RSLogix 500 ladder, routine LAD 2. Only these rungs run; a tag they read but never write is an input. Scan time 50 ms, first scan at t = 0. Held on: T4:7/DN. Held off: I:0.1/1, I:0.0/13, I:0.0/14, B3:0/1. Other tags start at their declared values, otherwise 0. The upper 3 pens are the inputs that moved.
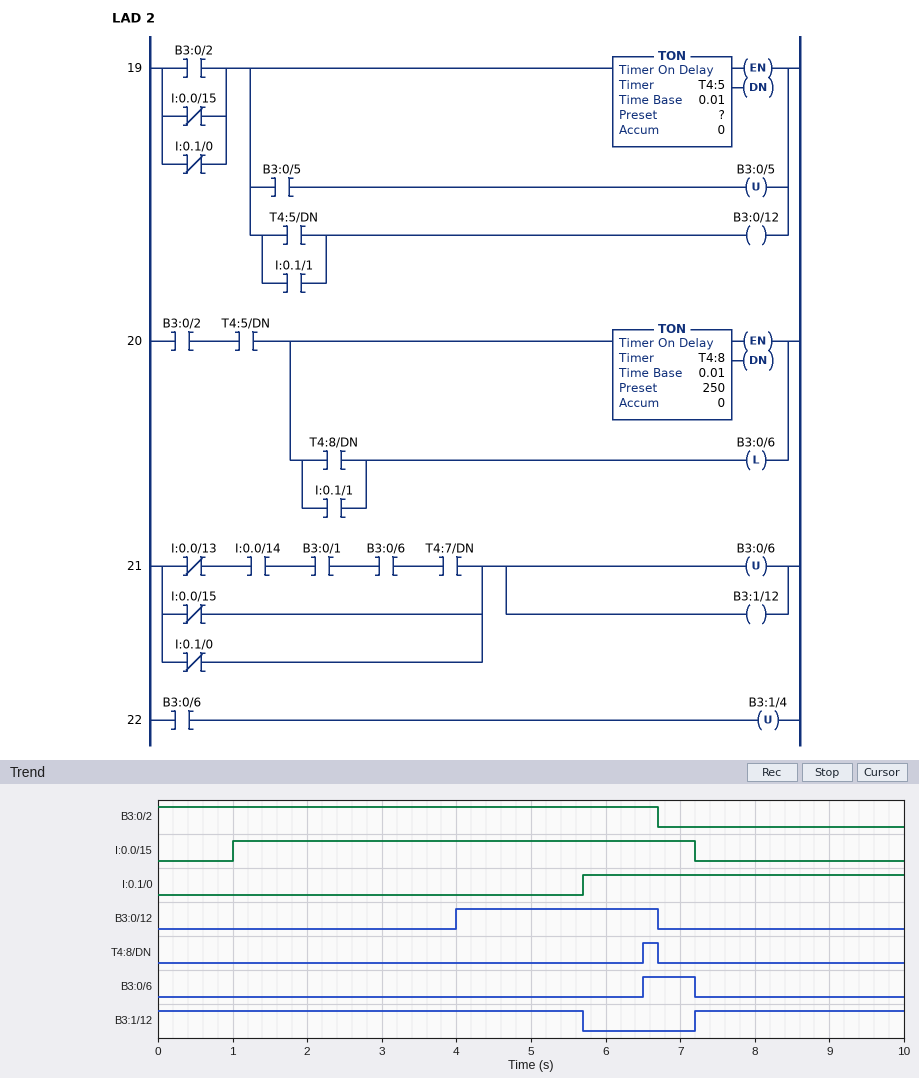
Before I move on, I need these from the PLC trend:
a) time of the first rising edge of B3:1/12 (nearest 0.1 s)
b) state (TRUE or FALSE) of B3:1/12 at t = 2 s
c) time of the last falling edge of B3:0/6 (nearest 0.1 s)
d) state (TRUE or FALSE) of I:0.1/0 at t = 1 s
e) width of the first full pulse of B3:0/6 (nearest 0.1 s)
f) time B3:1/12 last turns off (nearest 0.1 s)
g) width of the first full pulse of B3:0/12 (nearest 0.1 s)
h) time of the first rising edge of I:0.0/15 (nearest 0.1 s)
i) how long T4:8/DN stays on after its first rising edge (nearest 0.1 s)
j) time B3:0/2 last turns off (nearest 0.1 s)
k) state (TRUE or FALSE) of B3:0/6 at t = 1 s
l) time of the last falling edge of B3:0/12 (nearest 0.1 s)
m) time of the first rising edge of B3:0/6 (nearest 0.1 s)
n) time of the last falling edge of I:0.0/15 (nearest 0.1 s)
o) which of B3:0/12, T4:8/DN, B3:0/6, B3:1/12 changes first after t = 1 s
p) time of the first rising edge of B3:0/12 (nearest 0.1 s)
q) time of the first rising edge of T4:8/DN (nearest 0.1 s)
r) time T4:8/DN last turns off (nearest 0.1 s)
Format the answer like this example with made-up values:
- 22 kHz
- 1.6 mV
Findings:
- 7.2 s
- TRUE
- 7.2 s
- FALSE
- 0.7 s
- 5.7 s
- 2.7 s
- 1.0 s
- 0.2 s
- 6.7 s
- FALSE
- 6.7 s
- 6.5 s
- 7.2 s
- B3:0/12
- 4.0 s
- 6.5 s
- 6.7 s
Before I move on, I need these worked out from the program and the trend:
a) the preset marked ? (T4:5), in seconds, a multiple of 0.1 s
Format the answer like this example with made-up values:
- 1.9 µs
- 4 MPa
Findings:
- 4.0 s
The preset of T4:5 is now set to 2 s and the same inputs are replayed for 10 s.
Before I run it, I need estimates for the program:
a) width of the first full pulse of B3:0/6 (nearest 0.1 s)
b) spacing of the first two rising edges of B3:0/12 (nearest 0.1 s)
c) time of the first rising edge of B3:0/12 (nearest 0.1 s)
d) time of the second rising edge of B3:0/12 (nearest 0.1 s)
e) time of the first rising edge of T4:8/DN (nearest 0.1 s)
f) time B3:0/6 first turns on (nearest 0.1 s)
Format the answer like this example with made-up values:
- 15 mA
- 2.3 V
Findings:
- 1.5 s
- 7.2 s
- 2.0 s
- 9.2 s
- 4.5 s
- 5.7 s
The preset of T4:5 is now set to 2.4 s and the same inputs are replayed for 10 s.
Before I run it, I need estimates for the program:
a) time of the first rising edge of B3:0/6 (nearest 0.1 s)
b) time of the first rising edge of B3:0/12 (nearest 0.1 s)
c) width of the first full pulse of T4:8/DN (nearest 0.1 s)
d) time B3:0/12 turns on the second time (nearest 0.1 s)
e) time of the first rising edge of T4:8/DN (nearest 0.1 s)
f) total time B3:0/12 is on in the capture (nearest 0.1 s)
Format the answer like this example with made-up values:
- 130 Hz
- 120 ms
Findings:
- 5.7 s
- 2.4 s
- 1.8 s
- 9.6 s
- 4.9 s
- 4.7 s
